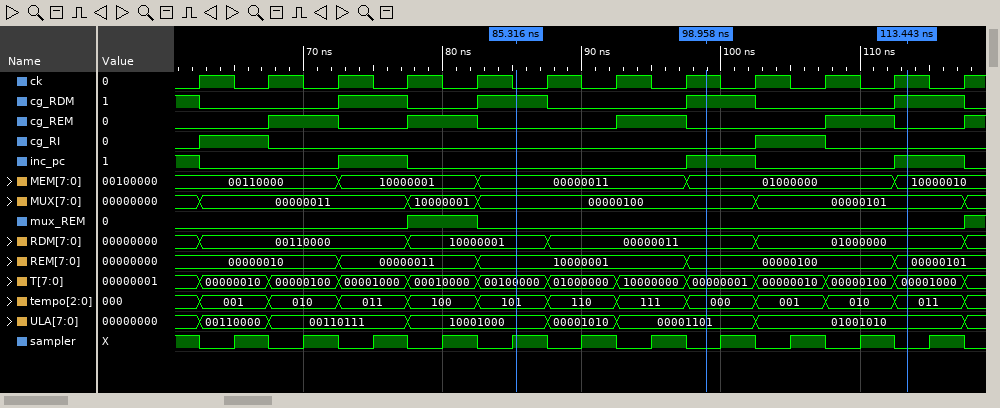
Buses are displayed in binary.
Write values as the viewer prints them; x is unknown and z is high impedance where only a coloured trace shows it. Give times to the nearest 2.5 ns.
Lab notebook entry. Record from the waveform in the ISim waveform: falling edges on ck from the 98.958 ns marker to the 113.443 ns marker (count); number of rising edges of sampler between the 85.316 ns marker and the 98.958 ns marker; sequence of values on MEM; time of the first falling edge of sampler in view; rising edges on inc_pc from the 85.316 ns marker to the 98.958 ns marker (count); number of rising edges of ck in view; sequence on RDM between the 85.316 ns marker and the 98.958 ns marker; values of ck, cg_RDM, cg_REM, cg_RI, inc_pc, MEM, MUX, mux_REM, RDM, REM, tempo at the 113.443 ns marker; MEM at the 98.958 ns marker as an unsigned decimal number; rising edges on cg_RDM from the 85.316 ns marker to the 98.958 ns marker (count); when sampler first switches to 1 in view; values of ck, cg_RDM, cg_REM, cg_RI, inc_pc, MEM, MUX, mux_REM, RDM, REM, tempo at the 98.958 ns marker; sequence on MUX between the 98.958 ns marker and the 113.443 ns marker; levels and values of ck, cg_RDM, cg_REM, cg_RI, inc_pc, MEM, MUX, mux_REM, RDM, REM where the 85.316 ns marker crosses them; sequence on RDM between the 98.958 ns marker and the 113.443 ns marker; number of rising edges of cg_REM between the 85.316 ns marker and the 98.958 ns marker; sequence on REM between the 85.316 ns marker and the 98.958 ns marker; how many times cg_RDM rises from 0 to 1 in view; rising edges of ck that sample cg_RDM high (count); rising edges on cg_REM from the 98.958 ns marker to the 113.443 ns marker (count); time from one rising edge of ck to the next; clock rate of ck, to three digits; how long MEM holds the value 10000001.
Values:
3
2
00110000, 10000001, 00000011, 01000000, 10000010
62.5 ns
1
12
10000001, 00000011
ck=1, cg_RDM=1, cg_REM=0, cg_RI=0, inc_pc=1, MEM=10000010, MUX=00000101, mux_REM=0, RDM=01000000, REM=00000101, tempo=011
64
1
65 ns
ck=1, cg_RDM=1, cg_REM=0, cg_RI=0, inc_pc=1, MEM=01000000, MUX=00000100, mux_REM=0, RDM=00000011, REM=00000100, tempo=000
00000100, 00000101
ck=0, cg_RDM=1, cg_REM=0, cg_RI=0, inc_pc=0, MEM=00000011, MUX=00000100, mux_REM=0, RDM=10000001, REM=10000001
00000011, 01000000
1
10000001, 00000100
4
5
1
5 ns
200 MHz
10 ns
